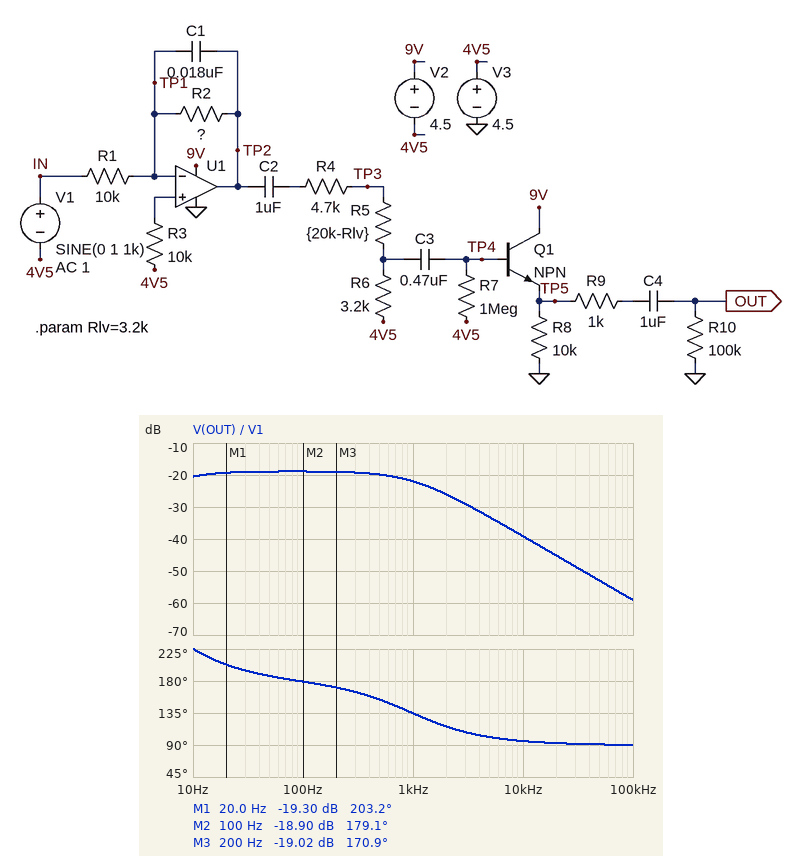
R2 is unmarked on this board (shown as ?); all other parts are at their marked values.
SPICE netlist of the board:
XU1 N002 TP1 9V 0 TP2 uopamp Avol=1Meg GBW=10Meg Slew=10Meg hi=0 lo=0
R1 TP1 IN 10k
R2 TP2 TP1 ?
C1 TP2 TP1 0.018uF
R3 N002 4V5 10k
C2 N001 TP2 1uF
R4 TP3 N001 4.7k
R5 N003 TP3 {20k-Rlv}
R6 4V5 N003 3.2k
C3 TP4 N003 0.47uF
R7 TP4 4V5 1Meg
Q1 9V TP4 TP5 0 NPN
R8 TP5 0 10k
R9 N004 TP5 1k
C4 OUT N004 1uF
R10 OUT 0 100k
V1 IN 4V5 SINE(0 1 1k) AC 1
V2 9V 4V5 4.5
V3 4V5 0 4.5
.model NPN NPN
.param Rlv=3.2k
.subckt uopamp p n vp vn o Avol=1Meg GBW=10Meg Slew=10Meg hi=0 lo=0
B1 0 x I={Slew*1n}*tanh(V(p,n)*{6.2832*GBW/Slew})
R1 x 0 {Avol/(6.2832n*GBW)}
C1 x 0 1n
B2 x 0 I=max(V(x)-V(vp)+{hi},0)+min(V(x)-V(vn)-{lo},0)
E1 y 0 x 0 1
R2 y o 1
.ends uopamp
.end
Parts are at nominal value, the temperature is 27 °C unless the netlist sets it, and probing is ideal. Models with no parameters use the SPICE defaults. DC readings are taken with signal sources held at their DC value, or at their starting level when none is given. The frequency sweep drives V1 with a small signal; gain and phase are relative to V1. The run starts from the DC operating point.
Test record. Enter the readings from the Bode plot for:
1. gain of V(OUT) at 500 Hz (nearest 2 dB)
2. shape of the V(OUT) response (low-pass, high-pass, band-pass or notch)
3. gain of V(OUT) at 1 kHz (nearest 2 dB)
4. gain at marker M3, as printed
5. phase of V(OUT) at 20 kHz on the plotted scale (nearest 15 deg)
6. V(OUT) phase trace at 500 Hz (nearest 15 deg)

-20 dB
low-pass
-22 dB
-19.02 dB
90 deg
150 deg
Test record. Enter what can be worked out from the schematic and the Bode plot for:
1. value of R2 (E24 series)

9.1 kΩ
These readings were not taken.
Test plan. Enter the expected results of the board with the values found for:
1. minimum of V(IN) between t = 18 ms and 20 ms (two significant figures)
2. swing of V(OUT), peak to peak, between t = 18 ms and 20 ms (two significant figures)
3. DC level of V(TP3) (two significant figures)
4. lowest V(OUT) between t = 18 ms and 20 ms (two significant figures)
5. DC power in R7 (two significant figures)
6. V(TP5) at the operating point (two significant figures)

3.5 V
160 mV
4.5 V
-79 mV
3.5 µW
1.9 V
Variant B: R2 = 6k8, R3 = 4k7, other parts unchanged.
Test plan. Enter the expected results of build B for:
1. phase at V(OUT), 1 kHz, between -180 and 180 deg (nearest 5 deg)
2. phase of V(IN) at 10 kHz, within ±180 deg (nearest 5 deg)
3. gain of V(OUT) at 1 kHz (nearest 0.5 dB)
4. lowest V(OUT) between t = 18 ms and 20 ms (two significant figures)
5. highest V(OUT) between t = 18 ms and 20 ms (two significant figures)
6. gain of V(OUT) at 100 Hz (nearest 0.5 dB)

145 deg
0 deg
-23.5 dB
-67 mV
68 mV
-21.5 dB
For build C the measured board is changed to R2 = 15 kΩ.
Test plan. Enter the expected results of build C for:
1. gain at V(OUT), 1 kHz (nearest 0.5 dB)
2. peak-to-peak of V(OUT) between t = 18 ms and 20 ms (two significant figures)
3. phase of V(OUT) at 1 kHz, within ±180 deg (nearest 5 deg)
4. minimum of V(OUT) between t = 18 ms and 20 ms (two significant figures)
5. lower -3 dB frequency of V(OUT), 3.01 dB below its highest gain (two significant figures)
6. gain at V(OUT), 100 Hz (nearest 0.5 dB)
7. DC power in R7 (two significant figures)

-20.5 dB
190 mV
120 deg
-95 mV
6.7 Hz
-14.5 dB
3.5 µW
